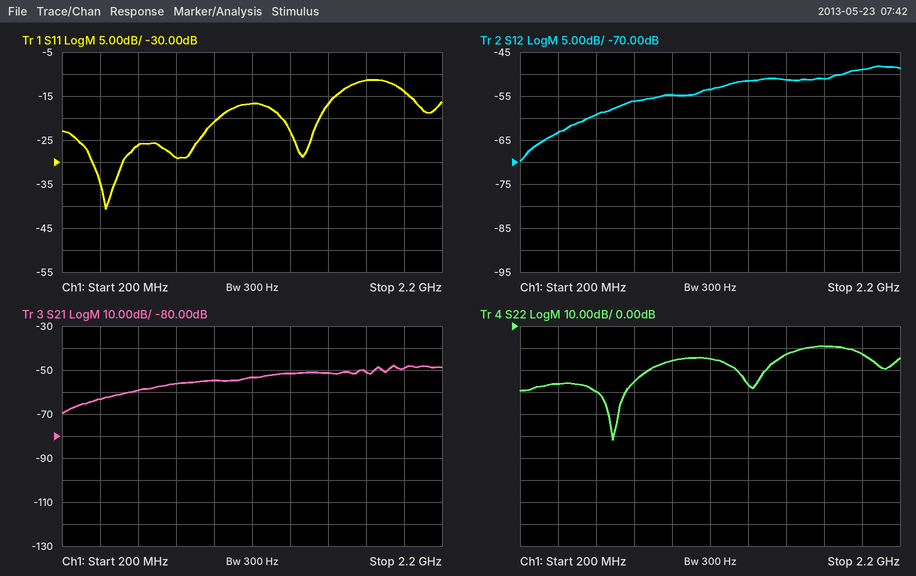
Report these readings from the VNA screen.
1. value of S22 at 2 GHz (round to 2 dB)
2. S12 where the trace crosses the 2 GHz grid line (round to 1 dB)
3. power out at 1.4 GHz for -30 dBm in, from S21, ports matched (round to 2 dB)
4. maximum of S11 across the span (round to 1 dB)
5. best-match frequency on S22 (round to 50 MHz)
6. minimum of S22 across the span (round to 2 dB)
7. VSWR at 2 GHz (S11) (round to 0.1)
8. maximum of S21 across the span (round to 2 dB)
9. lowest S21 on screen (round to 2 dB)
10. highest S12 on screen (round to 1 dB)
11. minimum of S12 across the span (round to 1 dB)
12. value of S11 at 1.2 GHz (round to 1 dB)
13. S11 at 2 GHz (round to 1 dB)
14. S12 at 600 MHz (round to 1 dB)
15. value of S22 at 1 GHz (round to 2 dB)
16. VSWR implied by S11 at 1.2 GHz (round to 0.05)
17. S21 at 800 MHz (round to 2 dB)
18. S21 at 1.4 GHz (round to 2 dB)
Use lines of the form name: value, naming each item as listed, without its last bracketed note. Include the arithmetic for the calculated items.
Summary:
value of S22 at 2 GHz: -12 dB
S12 where the trace crosses the 2 GHz grid line: -49 dB
power out at 1.4 GHz for -30 dBm in, from S21, ports matched: -30 dBm + (-52 dB) = -82 dBm
maximum of S11 across the span: -11 dB
best-match frequency on S22: 700 MHz
minimum of S22 across the span: -52 dB
VSWR at 2 GHz (S11): |Γ| = 10^(-14/20) = 0.1995; VSWR = (1 + 0.1995)/(1 − 0.1995) ≈ 1.5
maximum of S21 across the span: -48 dB
lowest S21 on screen: -70 dB
highest S12 on screen: -48 dB
minimum of S12 across the span: -70 dB
value of S11 at 1.2 GHz: -17 dB
S11 at 2 GHz: -14 dB
S12 at 600 MHz: -59 dB
value of S22 at 1 GHz: -16 dB
VSWR implied by S11 at 1.2 GHz: |Γ| = 10^(-17/20) = 0.1413; VSWR = (1 + 0.1413)/(1 − 0.1413) ≈ 1.33, so 1.35 to the nearest 0.05
S21 at 800 MHz: -56 dB
S21 at 1.4 GHz: -52 dB
